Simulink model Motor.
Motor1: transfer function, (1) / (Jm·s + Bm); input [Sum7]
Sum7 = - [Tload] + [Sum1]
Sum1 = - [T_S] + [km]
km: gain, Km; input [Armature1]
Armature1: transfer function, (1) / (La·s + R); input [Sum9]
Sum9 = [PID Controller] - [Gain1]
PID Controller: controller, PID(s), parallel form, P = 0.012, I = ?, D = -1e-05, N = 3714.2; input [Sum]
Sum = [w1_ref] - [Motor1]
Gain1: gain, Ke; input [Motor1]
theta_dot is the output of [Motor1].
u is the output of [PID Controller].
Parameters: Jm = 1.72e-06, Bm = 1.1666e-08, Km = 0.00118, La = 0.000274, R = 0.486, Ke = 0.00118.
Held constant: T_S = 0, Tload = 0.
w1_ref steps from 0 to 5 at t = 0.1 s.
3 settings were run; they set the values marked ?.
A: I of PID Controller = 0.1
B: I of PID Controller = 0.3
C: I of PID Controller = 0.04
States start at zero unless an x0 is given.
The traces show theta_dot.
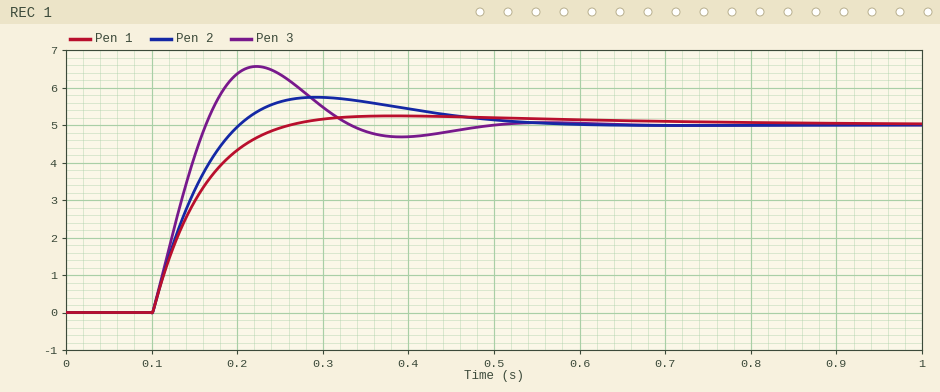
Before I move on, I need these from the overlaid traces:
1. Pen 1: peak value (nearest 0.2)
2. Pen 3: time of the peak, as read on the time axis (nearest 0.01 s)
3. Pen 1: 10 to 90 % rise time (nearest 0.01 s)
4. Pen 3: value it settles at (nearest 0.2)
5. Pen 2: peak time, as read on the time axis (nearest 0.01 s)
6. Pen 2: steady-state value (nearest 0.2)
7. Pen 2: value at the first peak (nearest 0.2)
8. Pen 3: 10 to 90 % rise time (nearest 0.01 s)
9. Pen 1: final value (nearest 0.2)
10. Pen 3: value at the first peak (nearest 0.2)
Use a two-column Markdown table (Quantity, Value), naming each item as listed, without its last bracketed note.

| Quantity | Value |
|---|---|
| Pen 1: peak value | 5.2 |
| Pen 3: time of the peak, as read on the time axis | 0.22 s |
| Pen 1: 10 to 90 % rise time | 0.10 s |
| Pen 3: value it settles at | 5.0 |
| Pen 2: peak time, as read on the time axis | 0.29 s |
| Pen 2: steady-state value | 5.0 |
| Pen 2: value at the first peak | 5.8 |
| Pen 3: 10 to 90 % rise time | 0.05 s |
| Pen 1: final value | 5.0 |
| Pen 3: value at the first peak | 6.6 |
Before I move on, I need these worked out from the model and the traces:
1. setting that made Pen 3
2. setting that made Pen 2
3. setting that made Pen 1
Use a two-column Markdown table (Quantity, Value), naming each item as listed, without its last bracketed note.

| Quantity | Value |
|---|---|
| setting that made Pen 3 | B |
| setting that made Pen 2 | A |
| setting that made Pen 1 | C |
